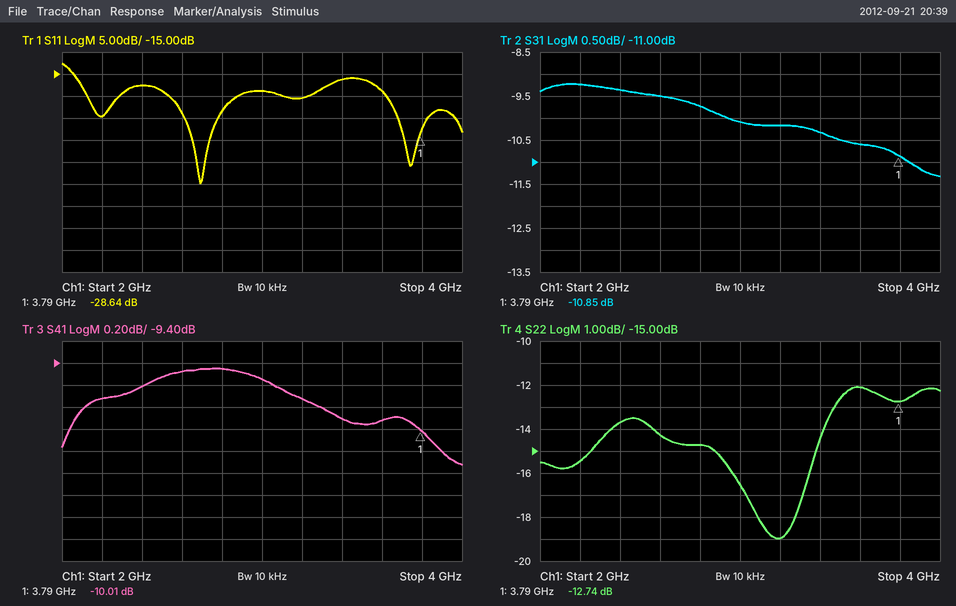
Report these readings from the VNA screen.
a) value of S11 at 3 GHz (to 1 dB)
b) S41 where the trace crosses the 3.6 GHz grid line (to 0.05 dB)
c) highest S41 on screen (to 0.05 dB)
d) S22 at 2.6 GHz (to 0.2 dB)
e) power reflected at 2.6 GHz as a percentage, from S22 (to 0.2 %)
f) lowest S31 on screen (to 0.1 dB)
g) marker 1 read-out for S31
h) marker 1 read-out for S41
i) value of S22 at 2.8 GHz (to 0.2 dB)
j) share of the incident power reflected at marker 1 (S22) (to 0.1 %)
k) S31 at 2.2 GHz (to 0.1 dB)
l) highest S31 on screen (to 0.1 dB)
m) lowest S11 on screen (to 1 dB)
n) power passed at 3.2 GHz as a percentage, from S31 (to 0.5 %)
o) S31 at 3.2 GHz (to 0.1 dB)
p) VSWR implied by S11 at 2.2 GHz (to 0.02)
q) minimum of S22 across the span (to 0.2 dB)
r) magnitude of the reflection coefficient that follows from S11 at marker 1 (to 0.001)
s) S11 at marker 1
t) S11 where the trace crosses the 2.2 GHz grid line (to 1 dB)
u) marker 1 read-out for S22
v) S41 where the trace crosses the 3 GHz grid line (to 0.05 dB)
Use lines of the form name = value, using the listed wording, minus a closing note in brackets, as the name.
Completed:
value of S11 at 3 GHz = -19 dB
S41 where the trace crosses the 3.6 GHz grid line = -9.90 dB
highest S41 on screen = -9.45 dB
S22 at 2.6 GHz = -14.2 dB
power reflected at 2.6 GHz as a percentage, from S22 = 3.8 %
lowest S31 on screen = -11.3 dB
marker 1 read-out for S31 = -10.85 dB
marker 1 read-out for S41 = -10.01 dB
value of S22 at 2.8 GHz = -14.8 dB
share of the incident power reflected at marker 1 (S22) = 5.3 %
S31 at 2.2 GHz = -9.2 dB
highest S31 on screen = -9.2 dB
lowest S11 on screen = -40 dB
power passed at 3.2 GHz as a percentage, from S31 = 9.5 %
S31 at 3.2 GHz = -10.2 dB
VSWR implied by S11 at 2.2 GHz = 1.12
minimum of S22 across the span = -19.0 dB
magnitude of the reflection coefficient that follows from S11 at marker 1 = 0.037
S11 at marker 1 = -28.64 dB
S11 where the trace crosses the 2.2 GHz grid line = -25 dB
marker 1 read-out for S22 = -12.74 dB
S41 where the trace crosses the 3 GHz grid line = -9.55 dB
